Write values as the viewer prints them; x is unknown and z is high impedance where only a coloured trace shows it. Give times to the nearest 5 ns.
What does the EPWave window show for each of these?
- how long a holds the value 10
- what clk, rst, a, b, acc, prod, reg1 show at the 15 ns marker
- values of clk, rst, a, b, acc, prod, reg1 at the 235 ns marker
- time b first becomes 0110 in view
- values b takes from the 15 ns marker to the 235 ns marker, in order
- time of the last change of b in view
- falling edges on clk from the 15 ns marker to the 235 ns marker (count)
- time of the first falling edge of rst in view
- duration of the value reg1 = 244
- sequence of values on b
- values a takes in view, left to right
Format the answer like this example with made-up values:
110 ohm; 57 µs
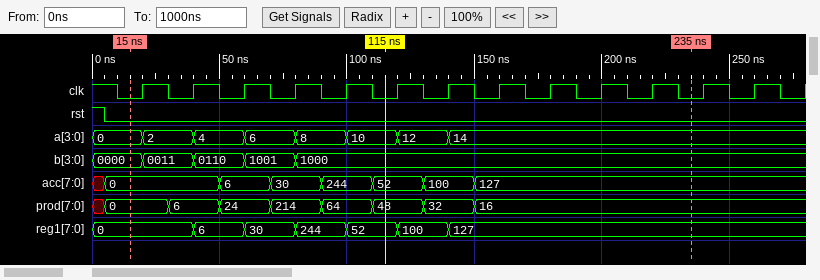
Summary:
20 ns; clk=0, rst=0, a=0, b=0000, acc=0, prod=0, reg1=0; clk=0, rst=0, a=14, b=1000, acc=127, prod=16, reg1=127; 40 ns; 0000, 0011, 0110, 1001, 1000; 80 ns; 11; 5 ns; 20 ns; 0000, 0011, 0110, 1001, 1000; 0, 2, 4, 6, 8, 10, 12, 14
